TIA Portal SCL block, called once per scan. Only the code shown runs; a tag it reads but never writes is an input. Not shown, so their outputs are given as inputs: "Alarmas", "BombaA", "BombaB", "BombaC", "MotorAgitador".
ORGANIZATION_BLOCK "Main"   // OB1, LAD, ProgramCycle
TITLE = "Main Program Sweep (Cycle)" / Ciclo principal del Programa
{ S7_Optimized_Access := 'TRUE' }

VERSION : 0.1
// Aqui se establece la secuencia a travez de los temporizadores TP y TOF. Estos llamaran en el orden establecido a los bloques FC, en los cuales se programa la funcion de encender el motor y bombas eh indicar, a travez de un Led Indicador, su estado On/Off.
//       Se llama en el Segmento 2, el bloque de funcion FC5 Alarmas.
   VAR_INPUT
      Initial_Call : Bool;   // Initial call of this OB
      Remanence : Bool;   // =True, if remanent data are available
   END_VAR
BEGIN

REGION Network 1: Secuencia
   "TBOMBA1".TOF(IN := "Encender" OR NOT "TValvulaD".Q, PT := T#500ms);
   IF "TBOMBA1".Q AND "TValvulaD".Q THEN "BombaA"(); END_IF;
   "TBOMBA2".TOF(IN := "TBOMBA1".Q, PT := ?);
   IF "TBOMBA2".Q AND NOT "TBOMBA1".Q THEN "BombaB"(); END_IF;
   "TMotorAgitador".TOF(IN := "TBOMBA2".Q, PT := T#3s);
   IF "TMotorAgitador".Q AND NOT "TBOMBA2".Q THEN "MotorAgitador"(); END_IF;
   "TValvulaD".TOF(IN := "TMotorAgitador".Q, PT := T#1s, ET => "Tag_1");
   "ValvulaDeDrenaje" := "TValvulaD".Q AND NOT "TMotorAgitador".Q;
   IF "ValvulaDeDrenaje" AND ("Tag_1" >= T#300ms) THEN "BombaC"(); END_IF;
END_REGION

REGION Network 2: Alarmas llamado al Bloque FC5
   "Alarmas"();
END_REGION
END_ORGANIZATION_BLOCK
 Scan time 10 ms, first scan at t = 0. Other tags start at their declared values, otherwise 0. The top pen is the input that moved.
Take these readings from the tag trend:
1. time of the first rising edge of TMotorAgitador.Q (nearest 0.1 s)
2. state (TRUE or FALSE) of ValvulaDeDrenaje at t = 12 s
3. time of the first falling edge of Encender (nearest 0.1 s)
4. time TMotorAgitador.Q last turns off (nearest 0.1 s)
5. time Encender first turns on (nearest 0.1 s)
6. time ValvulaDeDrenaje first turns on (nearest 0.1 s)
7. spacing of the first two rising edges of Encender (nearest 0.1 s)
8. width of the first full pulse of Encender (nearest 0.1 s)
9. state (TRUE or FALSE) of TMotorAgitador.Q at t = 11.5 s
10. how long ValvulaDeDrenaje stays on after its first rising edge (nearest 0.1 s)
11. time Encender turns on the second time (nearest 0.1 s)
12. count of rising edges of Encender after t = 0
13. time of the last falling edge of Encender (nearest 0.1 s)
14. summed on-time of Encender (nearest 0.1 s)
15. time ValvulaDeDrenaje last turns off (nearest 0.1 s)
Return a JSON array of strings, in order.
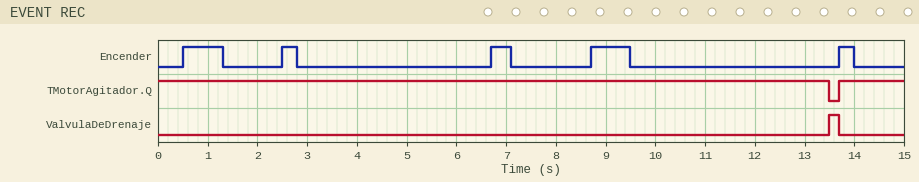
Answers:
["13.7 s", "FALSE", "1.3 s", "13.5 s", "0.5 s", "13.5 s", "2.0 s", "0.8 s", "TRUE", "0.2 s", "2.5 s", "5", "14.0 s", "2.6 s", "13.7 s"]
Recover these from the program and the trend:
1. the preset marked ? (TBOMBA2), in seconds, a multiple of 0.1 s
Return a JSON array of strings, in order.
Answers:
["0.5 s"]
